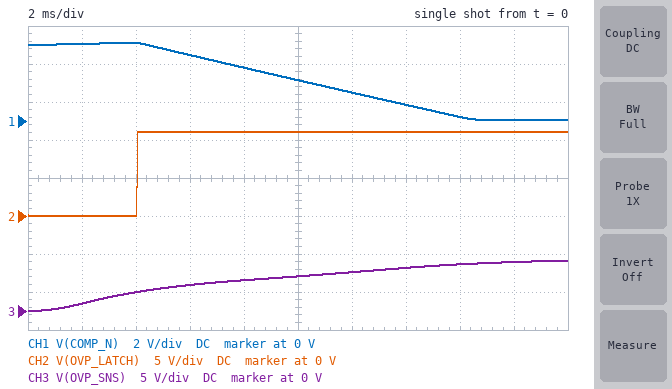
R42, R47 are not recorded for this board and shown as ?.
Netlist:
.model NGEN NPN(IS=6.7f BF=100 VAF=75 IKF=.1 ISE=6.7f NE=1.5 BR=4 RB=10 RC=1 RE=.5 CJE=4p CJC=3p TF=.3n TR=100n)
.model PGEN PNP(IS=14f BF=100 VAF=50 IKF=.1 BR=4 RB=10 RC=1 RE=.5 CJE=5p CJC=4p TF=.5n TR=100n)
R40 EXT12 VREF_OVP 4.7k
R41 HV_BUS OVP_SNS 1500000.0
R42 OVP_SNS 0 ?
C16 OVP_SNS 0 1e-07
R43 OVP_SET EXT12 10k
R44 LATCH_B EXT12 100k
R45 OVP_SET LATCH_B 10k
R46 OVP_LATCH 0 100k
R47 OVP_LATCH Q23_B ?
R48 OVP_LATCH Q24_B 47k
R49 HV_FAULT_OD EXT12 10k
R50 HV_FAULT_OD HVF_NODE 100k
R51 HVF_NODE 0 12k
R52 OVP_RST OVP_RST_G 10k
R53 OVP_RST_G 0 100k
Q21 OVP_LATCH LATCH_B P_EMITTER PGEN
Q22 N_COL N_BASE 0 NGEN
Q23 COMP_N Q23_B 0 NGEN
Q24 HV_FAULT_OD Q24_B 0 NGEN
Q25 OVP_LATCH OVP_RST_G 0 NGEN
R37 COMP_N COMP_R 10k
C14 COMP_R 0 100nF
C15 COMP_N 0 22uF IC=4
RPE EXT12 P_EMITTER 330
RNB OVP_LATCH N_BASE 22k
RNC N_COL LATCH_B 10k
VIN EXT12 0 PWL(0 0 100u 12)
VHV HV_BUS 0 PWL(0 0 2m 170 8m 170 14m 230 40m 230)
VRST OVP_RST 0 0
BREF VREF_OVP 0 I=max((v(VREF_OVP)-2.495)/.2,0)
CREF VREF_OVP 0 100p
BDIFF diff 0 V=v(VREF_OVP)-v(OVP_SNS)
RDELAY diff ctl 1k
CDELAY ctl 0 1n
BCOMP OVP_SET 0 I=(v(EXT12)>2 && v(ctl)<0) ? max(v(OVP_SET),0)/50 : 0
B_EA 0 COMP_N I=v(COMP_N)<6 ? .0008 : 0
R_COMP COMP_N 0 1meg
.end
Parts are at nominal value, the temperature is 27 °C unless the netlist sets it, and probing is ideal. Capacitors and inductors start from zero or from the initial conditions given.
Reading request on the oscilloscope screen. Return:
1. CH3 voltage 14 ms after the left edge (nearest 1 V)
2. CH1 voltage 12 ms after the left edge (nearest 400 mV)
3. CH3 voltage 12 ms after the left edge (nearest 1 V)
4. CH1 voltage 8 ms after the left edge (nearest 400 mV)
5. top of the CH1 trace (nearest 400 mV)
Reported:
6 V
1.6 V
5 V
2.8 V
4.0 V
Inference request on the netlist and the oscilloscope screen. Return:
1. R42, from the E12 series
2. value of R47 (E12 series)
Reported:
47 kΩ
120 kΩ
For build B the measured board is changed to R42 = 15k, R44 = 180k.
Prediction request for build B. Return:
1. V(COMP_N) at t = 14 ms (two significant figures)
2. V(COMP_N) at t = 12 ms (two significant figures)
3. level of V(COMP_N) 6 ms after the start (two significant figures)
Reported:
4.5 V
4.4 V
4.2 V
